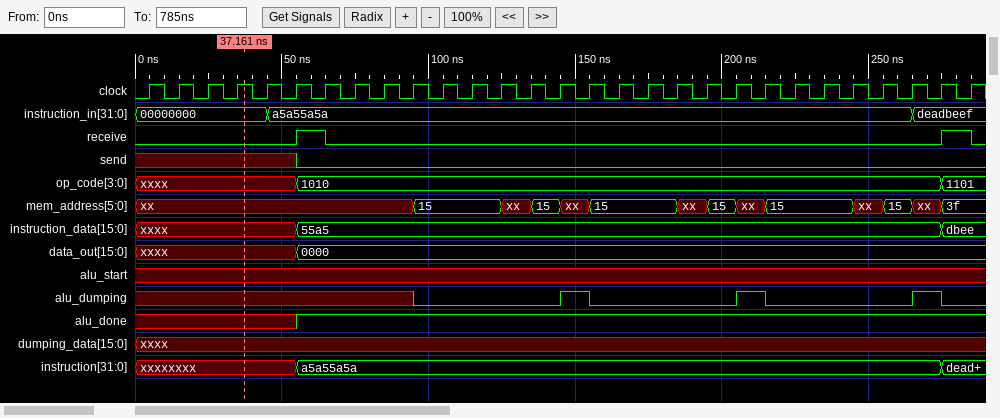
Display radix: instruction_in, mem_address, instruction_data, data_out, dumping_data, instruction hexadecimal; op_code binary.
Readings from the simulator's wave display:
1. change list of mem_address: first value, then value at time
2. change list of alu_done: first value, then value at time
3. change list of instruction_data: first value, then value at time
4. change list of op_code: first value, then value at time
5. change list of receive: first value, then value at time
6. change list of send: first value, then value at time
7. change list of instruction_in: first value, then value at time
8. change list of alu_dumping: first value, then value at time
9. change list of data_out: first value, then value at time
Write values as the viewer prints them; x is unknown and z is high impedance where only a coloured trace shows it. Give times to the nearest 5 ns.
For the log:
xx, 15 at 95 ns, xx at 125 ns, 15 at 135 ns, xx at 145 ns, 15 at 155 ns, xx at 185 ns, 15 at 195 ns, xx at 205 ns, 15 at 215 ns, xx at 245 ns, 15 at 255 ns, xx at 265 ns, 3f at 275 ns
x, 1 at 55 ns
xxxx, 55a5 at 55 ns, dbee at 275 ns
xxxx, 1010 at 55 ns, 1101 at 275 ns
0, 1 at 55 ns, 0 at 65 ns, 1 at 275 ns, 0 at 285 ns
x, 0 at 55 ns
00000000, a5a55a5a at 45 ns, deadbeef at 265 ns
x, 0 at 95 ns, 1 at 145 ns, 0 at 155 ns, 1 at 205 ns, 0 at 215 ns, 1 at 265 ns, 0 at 275 ns
xxxx, 0000 at 55 ns
